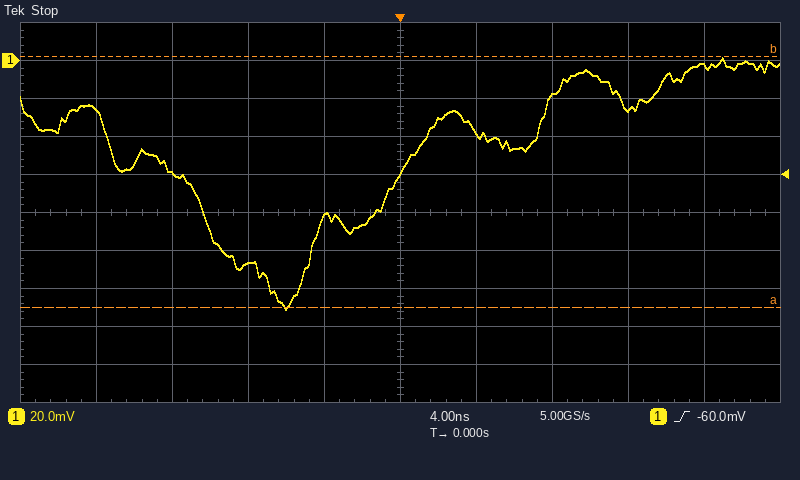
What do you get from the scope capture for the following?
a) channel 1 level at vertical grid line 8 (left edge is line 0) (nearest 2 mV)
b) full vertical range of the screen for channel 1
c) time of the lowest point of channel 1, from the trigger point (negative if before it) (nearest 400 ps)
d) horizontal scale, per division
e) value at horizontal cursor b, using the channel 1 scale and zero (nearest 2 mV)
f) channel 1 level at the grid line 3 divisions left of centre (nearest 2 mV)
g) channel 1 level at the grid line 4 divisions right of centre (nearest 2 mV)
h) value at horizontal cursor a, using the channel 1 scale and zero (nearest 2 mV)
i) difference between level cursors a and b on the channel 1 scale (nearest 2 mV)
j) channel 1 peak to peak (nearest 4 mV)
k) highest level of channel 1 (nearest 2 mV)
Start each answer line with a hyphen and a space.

- -26 mV
- 200 mV
- -6.0 ns
- 4 ns
- 2 mV
- -60 mV
- -4 mV
- -130 mV
- 132 mV
- 132 mV
- 2 mV
